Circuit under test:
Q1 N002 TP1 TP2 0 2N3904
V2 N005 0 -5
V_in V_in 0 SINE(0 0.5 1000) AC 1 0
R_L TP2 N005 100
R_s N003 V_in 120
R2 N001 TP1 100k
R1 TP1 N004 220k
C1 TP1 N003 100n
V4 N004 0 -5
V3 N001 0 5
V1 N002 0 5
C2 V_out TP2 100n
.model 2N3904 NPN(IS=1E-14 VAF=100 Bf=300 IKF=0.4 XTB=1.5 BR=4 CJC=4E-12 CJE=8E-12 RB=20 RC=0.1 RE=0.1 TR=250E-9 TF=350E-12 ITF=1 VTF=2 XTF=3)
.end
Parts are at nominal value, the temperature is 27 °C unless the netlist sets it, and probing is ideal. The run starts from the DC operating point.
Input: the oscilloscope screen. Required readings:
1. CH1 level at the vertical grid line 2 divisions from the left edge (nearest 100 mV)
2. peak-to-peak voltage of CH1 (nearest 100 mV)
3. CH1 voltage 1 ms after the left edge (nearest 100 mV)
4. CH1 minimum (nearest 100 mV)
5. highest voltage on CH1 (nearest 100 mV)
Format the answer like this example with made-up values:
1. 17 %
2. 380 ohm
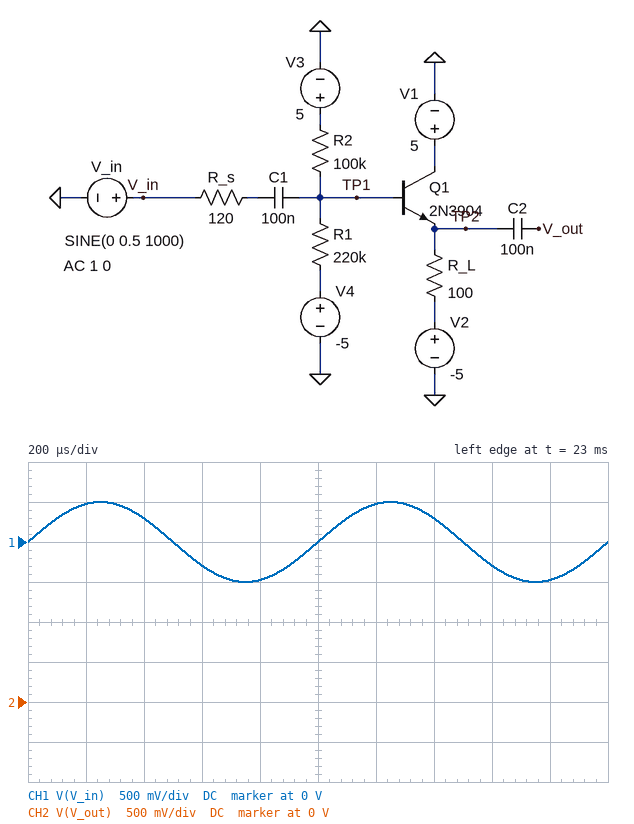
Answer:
1. 300 mV
2. 1.0 V
3. 0 V
4. -500 mV
5. 500 mV
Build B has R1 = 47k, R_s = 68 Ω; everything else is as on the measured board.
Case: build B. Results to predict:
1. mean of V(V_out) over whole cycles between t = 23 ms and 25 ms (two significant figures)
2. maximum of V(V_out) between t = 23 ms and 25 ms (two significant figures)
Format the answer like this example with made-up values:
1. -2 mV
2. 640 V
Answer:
1. -3.8 V
2. -3.3 V
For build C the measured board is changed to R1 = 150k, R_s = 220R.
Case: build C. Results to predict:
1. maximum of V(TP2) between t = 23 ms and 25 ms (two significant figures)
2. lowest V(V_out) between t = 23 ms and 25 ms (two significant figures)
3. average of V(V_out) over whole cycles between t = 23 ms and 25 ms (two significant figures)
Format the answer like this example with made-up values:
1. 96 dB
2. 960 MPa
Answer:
1. -2.7 V
2. -3.7 V
3. -3.2 V
